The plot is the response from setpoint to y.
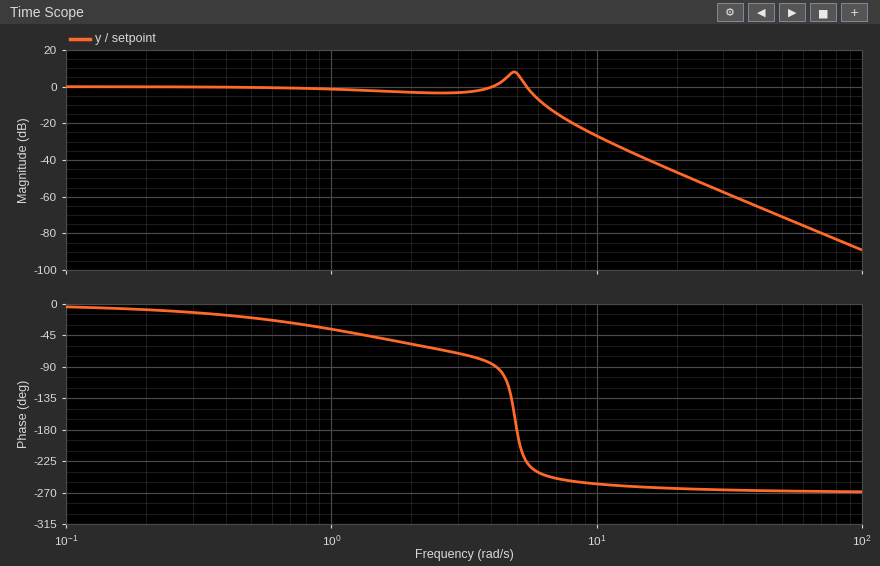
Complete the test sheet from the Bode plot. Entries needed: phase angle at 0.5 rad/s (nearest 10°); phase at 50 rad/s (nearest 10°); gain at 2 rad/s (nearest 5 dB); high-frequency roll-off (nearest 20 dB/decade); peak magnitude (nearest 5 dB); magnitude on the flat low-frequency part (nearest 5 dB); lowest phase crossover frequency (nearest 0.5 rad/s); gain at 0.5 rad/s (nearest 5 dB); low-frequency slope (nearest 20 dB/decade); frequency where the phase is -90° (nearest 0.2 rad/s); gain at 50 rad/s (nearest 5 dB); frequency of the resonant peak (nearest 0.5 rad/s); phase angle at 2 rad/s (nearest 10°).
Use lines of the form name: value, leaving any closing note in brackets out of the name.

phase angle at 0.5 rad/s: -20°
phase at 50 rad/s: -270°
gain at 2 rad/s: -5 dB
high-frequency roll-off: -60 dB/decade
peak magnitude: 10 dB
magnitude on the flat low-frequency part: 0 dB
lowest phase crossover frequency: 5.0 rad/s
gain at 0.5 rad/s: 0 dB
low-frequency slope: 0 dB/decade
frequency where the phase is -90°: 4.2 rad/s
gain at 50 rad/s: -70 dB
frequency of the resonant peak: 5.0 rad/s
phase angle at 2 rad/s: -60°
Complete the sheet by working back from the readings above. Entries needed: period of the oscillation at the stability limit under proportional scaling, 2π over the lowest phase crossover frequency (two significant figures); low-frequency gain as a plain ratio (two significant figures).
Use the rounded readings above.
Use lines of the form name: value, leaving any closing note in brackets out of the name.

period of the oscillation at the stability limit under proportional scaling, 2π over the lowest phase crossover frequency: 1.3 s
low-frequency gain as a plain ratio: 1.0
